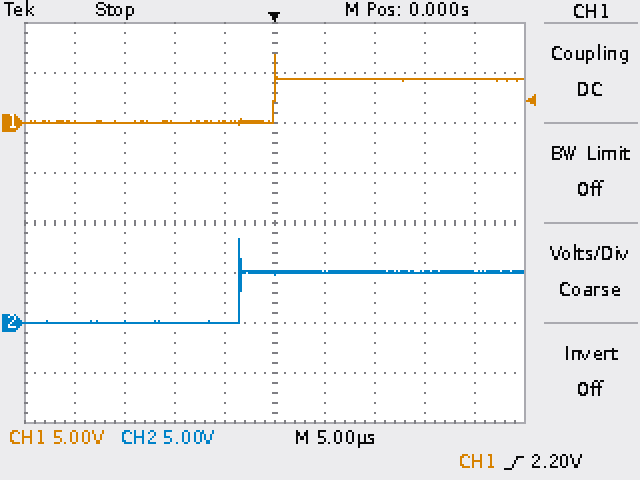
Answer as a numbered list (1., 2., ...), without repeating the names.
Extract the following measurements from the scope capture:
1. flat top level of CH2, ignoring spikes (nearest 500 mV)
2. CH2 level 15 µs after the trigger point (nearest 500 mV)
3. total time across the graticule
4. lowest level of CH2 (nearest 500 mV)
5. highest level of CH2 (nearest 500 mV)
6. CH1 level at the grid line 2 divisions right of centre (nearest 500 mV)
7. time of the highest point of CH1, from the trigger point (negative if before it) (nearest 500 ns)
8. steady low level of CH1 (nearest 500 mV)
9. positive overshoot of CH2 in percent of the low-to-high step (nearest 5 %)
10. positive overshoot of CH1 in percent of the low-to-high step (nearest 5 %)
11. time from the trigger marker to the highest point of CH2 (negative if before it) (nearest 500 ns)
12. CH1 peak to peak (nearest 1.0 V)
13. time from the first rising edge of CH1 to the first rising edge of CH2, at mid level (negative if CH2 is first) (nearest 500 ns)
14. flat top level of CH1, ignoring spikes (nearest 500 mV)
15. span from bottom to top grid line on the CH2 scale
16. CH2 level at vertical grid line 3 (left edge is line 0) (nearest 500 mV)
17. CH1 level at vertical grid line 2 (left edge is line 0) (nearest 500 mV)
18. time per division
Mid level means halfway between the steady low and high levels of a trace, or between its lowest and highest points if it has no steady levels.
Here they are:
1. 5.0 V
2. 5.0 V
3. 50 µs
4. 0.0 V
5. 8.5 V
6. 4.5 V
7. 0.0 µs
8. 0.0 V
9. 65 %
10. 55 %
11. -3.5 µs
12. 7.0 V
13. -3.5 µs
14. 4.5 V
15. 40 V
16. 0.0 V
17. 0.0 V
18. 5 µs
